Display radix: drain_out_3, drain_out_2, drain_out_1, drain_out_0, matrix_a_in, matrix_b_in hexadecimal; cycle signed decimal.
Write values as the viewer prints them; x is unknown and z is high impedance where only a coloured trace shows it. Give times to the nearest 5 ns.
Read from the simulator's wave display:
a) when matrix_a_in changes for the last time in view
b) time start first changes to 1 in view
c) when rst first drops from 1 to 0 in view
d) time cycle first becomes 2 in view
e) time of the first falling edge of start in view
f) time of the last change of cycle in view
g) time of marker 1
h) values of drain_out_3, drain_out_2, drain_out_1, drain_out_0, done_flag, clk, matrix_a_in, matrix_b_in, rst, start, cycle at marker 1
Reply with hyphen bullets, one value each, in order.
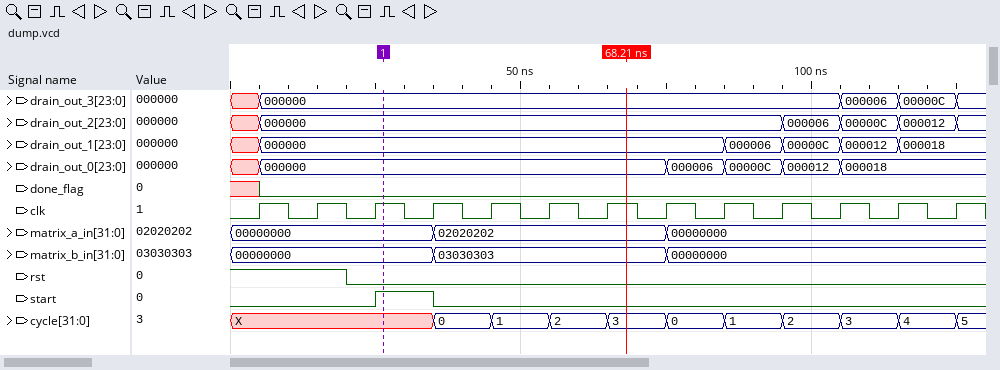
- 75 ns
- 25 ns
- 20 ns
- 55 ns
- 35 ns
- 125 ns
- 25 ns
- drain_out_3=000000, drain_out_2=000000, drain_out_1=000000, drain_out_0=000000, done_flag=0, clk=1, matrix_a_in=00000000, matrix_b_in=00000000, rst=0, start=1, cycle=X
